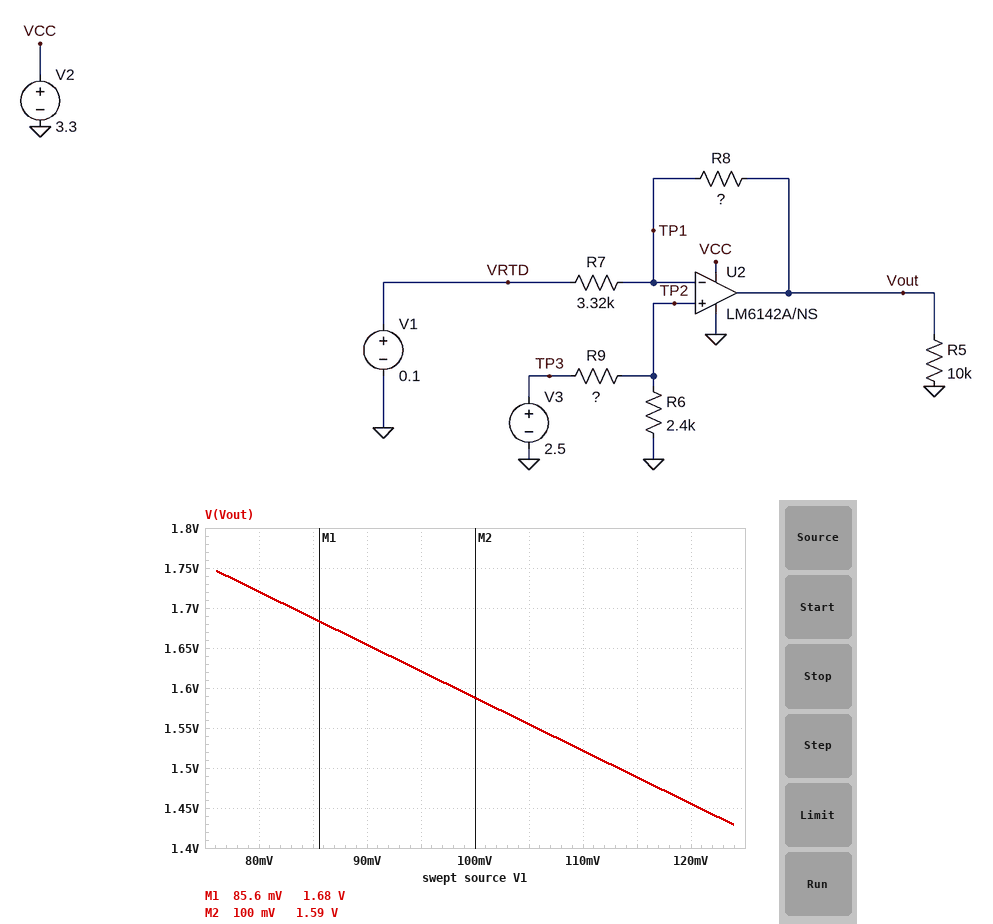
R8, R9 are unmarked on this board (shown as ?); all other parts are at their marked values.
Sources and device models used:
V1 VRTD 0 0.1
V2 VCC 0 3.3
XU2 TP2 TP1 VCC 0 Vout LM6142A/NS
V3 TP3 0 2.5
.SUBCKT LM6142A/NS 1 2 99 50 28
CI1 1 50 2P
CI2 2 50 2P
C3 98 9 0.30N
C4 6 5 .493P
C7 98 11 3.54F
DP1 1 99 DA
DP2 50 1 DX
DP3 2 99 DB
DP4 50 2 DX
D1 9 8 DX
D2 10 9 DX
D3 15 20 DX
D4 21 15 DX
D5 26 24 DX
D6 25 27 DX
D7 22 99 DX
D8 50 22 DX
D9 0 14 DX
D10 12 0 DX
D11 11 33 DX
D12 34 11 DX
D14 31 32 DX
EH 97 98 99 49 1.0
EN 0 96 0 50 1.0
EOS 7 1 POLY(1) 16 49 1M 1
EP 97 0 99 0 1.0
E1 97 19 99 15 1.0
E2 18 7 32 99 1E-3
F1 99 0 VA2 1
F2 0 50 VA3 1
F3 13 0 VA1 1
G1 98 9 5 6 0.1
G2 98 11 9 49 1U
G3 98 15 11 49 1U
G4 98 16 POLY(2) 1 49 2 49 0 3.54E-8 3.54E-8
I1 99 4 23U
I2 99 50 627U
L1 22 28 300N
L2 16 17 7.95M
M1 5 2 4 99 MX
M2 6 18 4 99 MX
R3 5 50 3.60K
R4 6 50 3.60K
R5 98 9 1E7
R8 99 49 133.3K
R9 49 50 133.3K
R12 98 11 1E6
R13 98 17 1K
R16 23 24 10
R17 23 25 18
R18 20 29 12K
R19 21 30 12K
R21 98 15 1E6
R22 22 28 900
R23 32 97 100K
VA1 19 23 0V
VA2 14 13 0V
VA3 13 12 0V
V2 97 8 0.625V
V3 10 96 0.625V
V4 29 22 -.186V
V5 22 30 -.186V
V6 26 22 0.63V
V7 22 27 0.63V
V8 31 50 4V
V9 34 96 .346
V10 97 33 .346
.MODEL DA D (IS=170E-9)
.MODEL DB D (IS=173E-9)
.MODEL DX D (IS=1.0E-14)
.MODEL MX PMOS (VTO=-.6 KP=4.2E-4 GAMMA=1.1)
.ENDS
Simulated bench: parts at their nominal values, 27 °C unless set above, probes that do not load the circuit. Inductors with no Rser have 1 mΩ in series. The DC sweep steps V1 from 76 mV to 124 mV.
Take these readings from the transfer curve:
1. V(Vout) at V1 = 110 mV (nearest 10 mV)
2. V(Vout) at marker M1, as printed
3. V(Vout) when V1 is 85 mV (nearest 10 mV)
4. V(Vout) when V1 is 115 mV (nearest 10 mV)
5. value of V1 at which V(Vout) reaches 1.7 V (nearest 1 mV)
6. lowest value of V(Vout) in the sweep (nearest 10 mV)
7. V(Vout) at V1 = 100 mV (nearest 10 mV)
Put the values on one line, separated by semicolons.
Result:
1.52 V; 1.68 V; 1.69 V; 1.49 V; 83 mV; 1.43 V; 1.59 V
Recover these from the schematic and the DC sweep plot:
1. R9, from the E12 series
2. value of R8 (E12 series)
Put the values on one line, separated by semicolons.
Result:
18 kΩ; 22 kΩ
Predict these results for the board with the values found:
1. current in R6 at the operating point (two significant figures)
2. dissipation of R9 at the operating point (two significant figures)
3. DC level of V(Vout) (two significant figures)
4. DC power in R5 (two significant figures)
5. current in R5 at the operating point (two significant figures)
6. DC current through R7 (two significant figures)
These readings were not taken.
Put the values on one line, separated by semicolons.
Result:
120 µA; 270 µW; 1.6 V; 250 µW; 160 µA; 59 µA
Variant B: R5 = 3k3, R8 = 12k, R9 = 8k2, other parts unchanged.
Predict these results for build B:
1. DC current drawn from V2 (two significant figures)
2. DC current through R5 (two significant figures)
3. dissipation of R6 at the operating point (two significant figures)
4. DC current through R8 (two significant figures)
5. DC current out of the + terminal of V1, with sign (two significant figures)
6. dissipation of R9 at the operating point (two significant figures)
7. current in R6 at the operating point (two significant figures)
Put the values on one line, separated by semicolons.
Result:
1.5 mA; 680 µA; 130 µW; 140 µA; -140 µA; 460 µW; 240 µA
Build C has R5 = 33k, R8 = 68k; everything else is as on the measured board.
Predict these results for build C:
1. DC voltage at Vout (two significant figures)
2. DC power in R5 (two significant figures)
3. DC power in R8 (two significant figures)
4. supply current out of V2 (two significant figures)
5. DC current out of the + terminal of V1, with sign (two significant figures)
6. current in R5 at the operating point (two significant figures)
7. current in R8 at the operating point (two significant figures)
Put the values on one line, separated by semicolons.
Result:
3.3 V; 330 µW; 140 µW; 810 µA; -45 µA; 100 µA; 45 µA
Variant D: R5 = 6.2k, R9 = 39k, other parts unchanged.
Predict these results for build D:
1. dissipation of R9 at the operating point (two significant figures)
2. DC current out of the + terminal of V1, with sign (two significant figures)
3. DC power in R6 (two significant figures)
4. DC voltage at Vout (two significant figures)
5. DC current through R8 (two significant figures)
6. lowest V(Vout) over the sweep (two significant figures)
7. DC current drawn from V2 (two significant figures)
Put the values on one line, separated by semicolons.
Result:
140 µW; -14 µA; 8.8 µW; 450 mV; 14 µA; 290 mV; 750 µA
